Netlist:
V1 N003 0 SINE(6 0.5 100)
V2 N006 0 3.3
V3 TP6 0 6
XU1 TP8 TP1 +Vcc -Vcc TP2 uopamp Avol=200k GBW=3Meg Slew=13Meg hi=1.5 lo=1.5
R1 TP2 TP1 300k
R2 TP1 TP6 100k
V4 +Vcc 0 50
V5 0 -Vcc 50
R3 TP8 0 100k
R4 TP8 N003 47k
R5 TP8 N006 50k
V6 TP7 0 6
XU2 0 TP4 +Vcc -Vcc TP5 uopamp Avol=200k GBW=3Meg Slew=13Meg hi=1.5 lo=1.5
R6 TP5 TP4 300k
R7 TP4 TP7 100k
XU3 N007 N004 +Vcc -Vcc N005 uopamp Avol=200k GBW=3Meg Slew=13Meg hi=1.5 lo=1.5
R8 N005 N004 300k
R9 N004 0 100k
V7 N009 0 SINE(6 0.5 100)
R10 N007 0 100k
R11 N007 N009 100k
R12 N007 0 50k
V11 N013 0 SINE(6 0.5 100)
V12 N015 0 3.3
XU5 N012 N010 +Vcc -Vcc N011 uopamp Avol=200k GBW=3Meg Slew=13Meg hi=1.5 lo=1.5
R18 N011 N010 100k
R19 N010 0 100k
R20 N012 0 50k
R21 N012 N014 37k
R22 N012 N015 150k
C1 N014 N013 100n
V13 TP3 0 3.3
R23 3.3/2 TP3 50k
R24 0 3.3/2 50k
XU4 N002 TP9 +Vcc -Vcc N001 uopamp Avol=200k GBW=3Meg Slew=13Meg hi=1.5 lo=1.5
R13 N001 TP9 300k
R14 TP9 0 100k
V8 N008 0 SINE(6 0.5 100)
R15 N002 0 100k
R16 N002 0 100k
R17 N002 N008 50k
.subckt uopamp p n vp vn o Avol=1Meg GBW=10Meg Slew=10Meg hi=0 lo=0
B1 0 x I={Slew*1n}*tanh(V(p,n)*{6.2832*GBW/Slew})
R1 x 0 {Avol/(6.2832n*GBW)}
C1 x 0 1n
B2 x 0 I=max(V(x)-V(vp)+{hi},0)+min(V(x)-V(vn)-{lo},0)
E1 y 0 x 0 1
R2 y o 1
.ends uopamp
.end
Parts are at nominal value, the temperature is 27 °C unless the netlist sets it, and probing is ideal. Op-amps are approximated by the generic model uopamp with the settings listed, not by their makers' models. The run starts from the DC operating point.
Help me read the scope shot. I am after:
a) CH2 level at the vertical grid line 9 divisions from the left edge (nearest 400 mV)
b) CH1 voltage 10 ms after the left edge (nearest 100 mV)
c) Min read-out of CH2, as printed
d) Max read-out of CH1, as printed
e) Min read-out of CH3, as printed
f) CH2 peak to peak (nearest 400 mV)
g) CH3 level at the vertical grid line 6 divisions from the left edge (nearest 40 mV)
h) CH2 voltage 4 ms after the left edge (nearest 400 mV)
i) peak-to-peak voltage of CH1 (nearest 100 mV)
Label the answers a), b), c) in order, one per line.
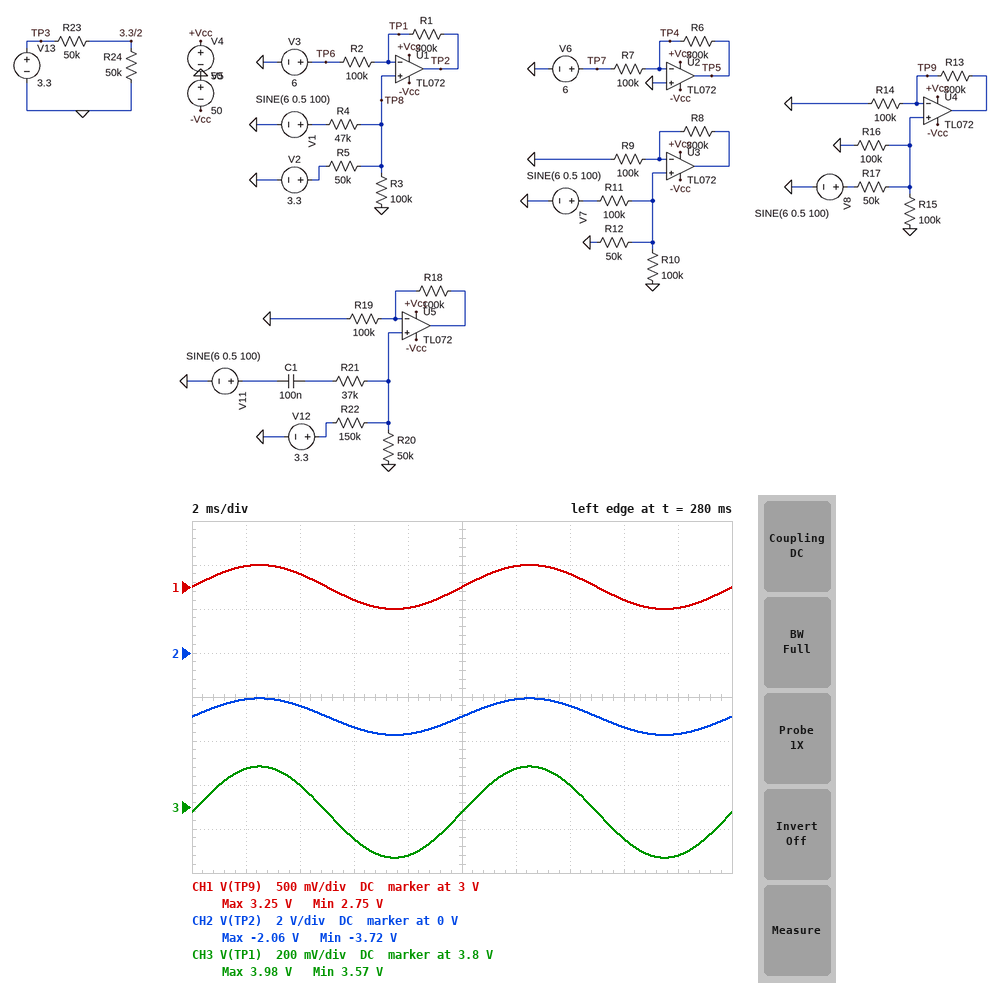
a) -3.6 V
b) 3.0 V
c) -3.72 V
d) 3.25 V
e) 3.57 V
f) 1.6 V
g) 3.96 V
h) -2.4 V
i) 500 mV
